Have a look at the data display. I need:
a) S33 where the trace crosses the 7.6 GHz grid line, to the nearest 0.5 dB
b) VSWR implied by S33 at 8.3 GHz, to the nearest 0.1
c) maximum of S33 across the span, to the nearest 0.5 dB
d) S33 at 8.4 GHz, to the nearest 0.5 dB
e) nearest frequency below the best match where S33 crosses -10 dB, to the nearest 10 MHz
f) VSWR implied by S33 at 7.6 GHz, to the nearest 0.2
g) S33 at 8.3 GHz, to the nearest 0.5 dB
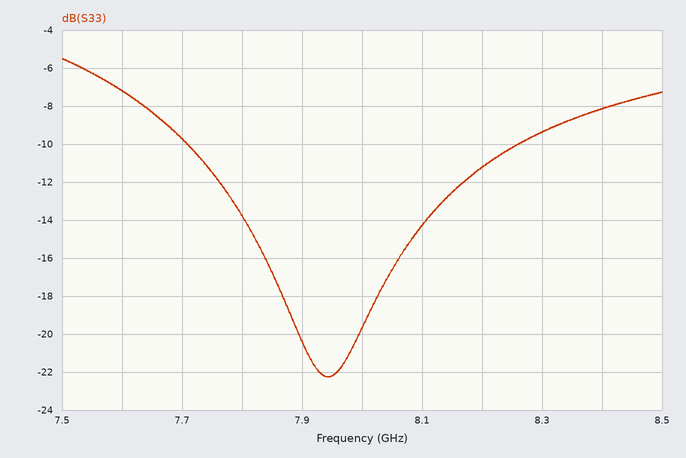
-7.0 dB
2.0
-5.5 dB
-8.0 dB
7.71 GHz
2.6
-9.5 dB
